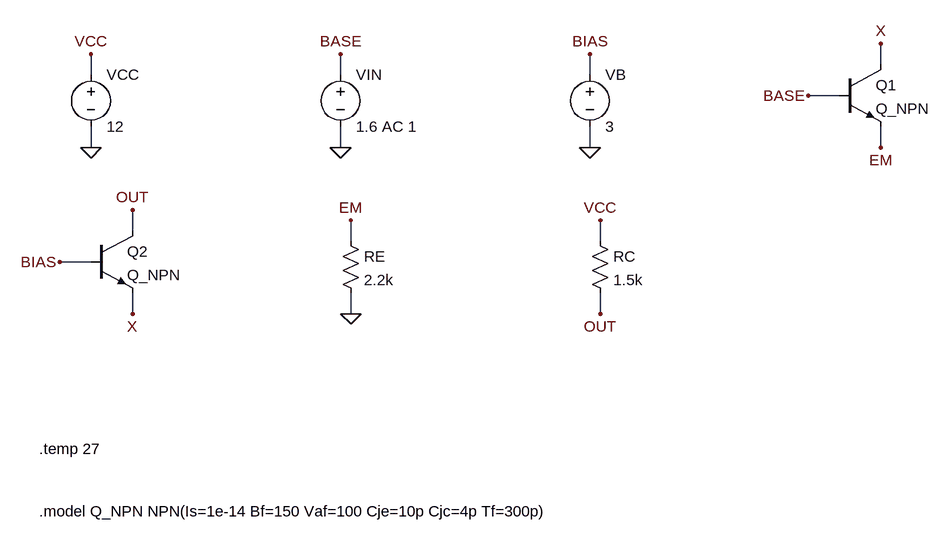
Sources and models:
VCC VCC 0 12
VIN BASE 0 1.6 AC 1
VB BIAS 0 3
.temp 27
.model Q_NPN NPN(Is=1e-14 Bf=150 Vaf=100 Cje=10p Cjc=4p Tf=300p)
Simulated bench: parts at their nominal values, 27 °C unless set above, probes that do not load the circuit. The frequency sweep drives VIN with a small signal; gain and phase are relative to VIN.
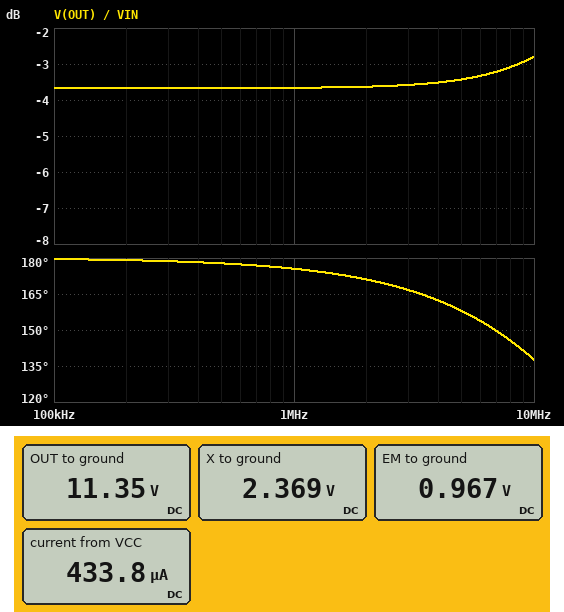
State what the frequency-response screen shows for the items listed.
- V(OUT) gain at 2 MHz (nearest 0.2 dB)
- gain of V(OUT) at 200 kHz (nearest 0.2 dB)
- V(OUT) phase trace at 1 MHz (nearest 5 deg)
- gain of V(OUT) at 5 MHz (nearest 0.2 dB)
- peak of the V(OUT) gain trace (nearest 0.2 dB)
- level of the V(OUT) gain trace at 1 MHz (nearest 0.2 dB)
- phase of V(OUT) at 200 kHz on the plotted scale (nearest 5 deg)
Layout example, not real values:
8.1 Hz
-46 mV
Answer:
-3.6 dB
-3.6 dB
175 deg
-3.4 dB
-2.8 dB
-3.6 dB
180 deg
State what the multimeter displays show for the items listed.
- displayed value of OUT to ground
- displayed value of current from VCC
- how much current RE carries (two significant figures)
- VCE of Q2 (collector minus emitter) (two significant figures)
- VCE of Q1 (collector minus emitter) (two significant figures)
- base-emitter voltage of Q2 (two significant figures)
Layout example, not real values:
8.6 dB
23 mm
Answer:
11.35 V
433.8 µA
440 µA
9.0 V
1.4 V
630 mV
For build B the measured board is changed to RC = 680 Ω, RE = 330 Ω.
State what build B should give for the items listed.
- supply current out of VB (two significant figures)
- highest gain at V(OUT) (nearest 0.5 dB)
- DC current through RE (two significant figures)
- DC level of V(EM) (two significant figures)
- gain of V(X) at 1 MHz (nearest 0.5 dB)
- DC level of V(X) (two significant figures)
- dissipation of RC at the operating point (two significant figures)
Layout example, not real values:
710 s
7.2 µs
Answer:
17 µA
6.0 dB
2.8 mA
920 mV
-31.0 dB
2.3 V
5.1 mW
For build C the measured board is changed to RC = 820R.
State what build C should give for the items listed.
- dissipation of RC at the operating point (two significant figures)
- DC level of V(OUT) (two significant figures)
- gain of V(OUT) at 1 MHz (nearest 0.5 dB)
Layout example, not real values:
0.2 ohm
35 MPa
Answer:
150 µW
12 V
-9.0 dB
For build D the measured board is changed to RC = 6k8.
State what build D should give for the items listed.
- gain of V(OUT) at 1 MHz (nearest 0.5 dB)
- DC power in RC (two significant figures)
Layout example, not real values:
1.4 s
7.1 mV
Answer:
9.5 dB
1.3 mW
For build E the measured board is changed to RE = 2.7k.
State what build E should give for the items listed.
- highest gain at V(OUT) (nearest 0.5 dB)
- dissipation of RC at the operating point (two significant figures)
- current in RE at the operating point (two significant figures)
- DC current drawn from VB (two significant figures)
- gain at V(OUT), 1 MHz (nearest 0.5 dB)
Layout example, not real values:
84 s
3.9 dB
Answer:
2.0 dB
190 µW
360 µA
2.2 µA
-5.5 dB
